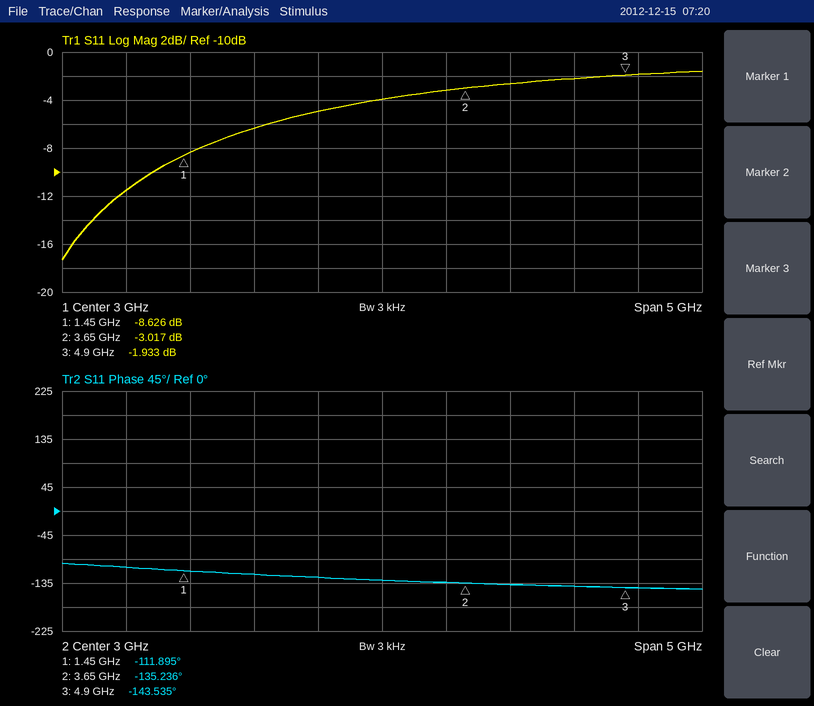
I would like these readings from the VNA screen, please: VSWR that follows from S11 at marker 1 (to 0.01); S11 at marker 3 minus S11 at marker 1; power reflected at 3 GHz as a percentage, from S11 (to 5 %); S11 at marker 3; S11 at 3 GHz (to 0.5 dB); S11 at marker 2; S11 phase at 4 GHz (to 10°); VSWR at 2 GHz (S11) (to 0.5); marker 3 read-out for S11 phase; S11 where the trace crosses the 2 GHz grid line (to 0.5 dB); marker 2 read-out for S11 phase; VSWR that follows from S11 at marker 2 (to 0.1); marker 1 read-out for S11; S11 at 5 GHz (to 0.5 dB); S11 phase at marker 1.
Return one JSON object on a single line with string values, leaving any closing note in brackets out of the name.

{"VSWR that follows from S11 at marker 1": "2.18", "S11 at marker 3 minus S11 at marker 1": "6.693 dB", "power reflected at 3 GHz as a percentage, from S11": "40 %", "S11 at marker 3": "-1.933 dB", "S11 at 3 GHz": "-4.0 dB", "S11 at marker 2": "-3.017 dB", "S11 phase at 4 GHz": "-140°", "VSWR at 2 GHz (S11)": "3.0", "marker 3 read-out for S11 phase": "-143.535°", "S11 where the trace crosses the 2 GHz grid line": "-6.5 dB", "marker 2 read-out for S11 phase": "-135.236°", "VSWR that follows from S11 at marker 2": "5.8", "marker 1 read-out for S11": "-8.626 dB", "S11 at 5 GHz": "-2.0 dB", "S11 phase at marker 1": "-111.895°"}
